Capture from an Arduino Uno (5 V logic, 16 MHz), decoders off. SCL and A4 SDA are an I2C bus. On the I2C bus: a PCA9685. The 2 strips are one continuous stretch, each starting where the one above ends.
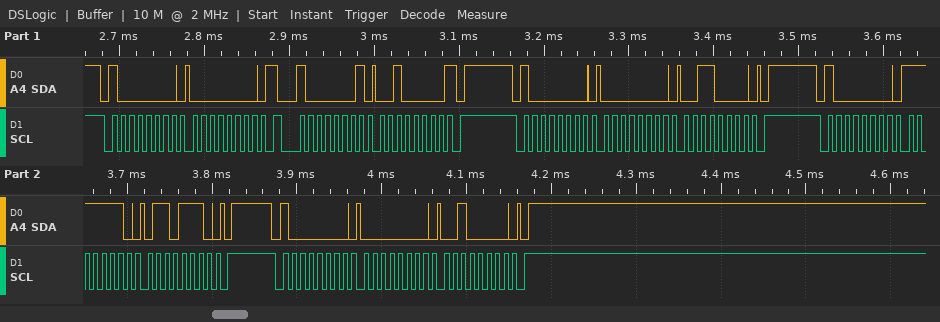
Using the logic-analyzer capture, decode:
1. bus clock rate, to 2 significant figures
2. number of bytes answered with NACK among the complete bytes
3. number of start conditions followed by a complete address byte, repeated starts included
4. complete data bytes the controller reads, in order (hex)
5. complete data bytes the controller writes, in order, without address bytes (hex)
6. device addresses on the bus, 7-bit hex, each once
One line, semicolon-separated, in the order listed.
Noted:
100 kHz; 1; 5; 20; 00 00 30 FE 6E 00 20; 0x40
